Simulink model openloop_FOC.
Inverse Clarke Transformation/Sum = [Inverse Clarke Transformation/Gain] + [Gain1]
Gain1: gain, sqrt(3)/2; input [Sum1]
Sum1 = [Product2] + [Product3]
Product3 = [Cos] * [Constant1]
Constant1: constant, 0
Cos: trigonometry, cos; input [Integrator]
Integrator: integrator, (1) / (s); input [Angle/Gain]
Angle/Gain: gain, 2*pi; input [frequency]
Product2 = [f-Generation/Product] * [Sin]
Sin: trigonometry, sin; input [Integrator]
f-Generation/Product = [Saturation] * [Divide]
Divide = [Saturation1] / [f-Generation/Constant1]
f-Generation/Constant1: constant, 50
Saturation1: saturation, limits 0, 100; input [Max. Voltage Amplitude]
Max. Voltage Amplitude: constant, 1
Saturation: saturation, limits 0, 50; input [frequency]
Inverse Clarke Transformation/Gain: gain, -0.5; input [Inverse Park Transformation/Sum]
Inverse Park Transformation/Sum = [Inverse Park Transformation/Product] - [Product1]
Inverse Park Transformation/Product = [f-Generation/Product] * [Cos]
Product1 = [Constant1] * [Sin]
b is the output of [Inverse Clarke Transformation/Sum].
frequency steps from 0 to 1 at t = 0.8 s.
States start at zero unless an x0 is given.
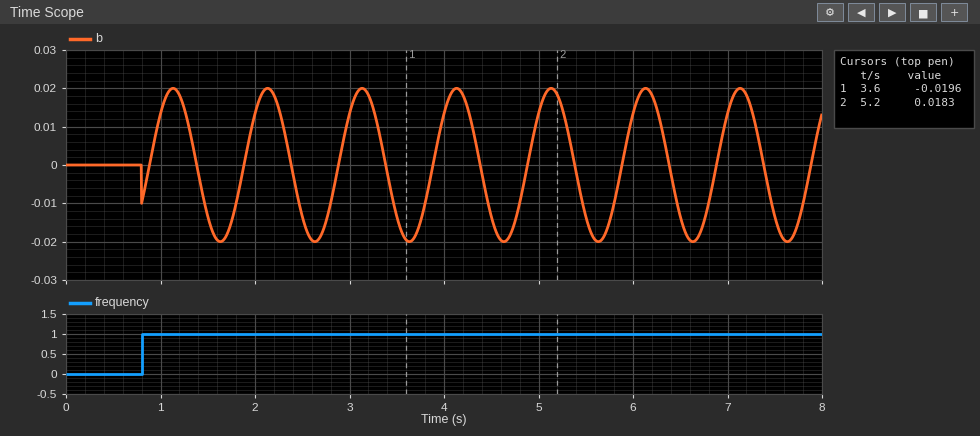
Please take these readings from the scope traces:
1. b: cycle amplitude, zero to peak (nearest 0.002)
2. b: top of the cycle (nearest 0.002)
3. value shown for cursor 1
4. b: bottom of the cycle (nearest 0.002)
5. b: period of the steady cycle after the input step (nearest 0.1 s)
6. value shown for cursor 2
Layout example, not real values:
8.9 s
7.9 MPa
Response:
0.020
0.020
-0.0196
-0.020
1.0 s
0.0183
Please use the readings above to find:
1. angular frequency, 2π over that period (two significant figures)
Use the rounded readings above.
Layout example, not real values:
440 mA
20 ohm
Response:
6.3 rad/s
